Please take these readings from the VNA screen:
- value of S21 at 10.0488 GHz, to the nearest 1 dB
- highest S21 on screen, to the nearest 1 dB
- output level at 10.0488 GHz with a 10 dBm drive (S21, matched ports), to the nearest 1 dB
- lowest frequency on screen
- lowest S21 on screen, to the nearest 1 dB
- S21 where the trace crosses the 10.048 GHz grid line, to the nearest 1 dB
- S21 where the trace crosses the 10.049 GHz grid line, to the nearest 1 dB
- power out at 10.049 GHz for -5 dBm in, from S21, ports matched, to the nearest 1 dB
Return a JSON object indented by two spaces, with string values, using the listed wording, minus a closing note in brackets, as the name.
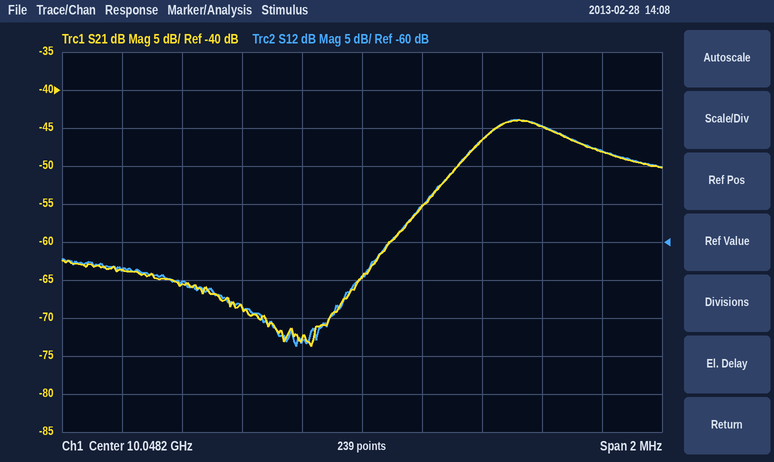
{
  "value of S21 at 10.0488 GHz, to the nearest 1 dB": "-45 dB",
  "highest S21 on screen, to the nearest 1 dB": "-44 dB",
  "output level at 10.0488 GHz with a 10 dBm drive (S21, matched ports), to the nearest 1 dB": "-35 dBm",
  "lowest frequency on screen": "10.0472 GHz",
  "lowest S21 on screen, to the nearest 1 dB": "-74 dB",
  "S21 where the trace crosses the 10.048 GHz grid line, to the nearest 1 dB": "-73 dB",
  "S21 where the trace crosses the 10.049 GHz grid line, to the nearest 1 dB": "-48 dB",
  "power out at 10.049 GHz for -5 dBm in, from S21, ports matched, to the nearest 1 dB": "-53 dBm"
}
